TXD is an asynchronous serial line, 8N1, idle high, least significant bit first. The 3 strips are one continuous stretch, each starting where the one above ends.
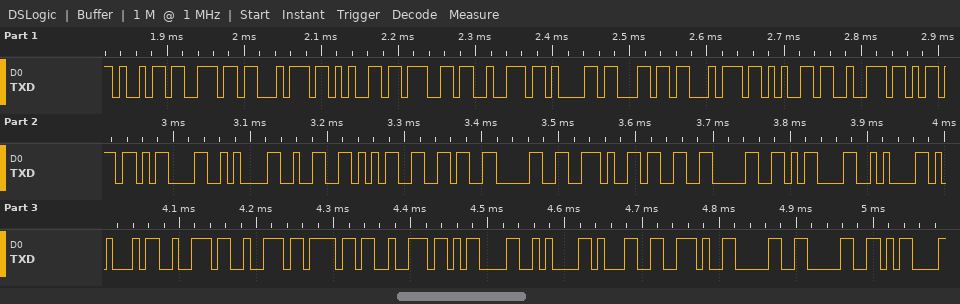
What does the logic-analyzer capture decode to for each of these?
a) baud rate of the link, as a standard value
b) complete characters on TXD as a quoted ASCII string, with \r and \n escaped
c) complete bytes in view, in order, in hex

115200 baud
"integralterm\r\n2560.30\r\nError\r\n1.00\r"
0x69 0x6E 0x74 0x65 0x67 0x72 0x61 0x6C 0x74 0x65 0x72 0x6D 0x0D 0x0A 0x32 0x35 0x36 0x30 0x2E 0x33 0x30 0x0D 0x0A 0x45 0x72 0x72 0x6F 0x72 0x0D 0x0A 0x31 0x2E 0x30 0x30 0x0D
